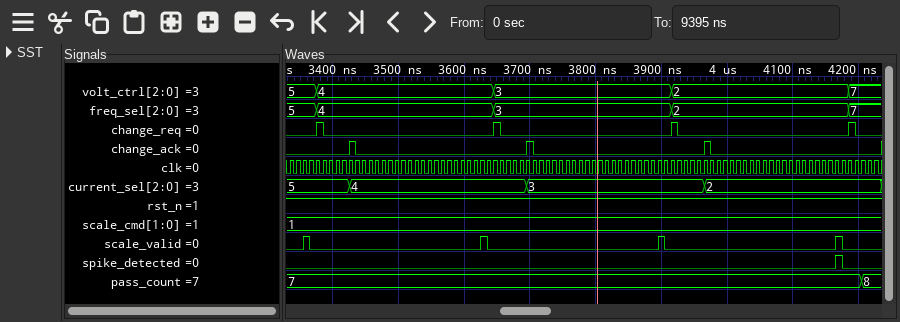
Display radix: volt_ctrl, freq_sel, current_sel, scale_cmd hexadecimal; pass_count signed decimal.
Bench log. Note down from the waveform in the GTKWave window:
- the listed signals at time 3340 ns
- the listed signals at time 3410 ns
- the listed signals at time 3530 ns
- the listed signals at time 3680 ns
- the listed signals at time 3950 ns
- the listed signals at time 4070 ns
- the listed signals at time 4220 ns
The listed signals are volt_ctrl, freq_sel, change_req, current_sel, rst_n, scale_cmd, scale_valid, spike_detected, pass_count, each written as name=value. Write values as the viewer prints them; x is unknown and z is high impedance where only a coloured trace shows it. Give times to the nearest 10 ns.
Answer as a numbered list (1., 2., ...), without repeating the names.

1. volt_ctrl=5, freq_sel=5, change_req=0, current_sel=5, rst_n=1, scale_cmd=1, scale_valid=0, spike_detected=0, pass_count=7
2. volt_ctrl=4, freq_sel=4, change_req=0, current_sel=5, rst_n=1, scale_cmd=1, scale_valid=0, spike_detected=0, pass_count=7
3. volt_ctrl=4, freq_sel=4, change_req=0, current_sel=4, rst_n=1, scale_cmd=1, scale_valid=0, spike_detected=0, pass_count=7
4. volt_ctrl=3, freq_sel=3, change_req=0, current_sel=4, rst_n=1, scale_cmd=1, scale_valid=0, spike_detected=0, pass_count=7
5. volt_ctrl=2, freq_sel=2, change_req=0, current_sel=3, rst_n=1, scale_cmd=1, scale_valid=0, spike_detected=0, pass_count=7
6. volt_ctrl=2, freq_sel=2, change_req=0, current_sel=2, rst_n=1, scale_cmd=1, scale_valid=0, spike_detected=0, pass_count=7
7. volt_ctrl=7, freq_sel=7, change_req=0, current_sel=2, rst_n=1, scale_cmd=1, scale_valid=0, spike_detected=0, pass_count=8
